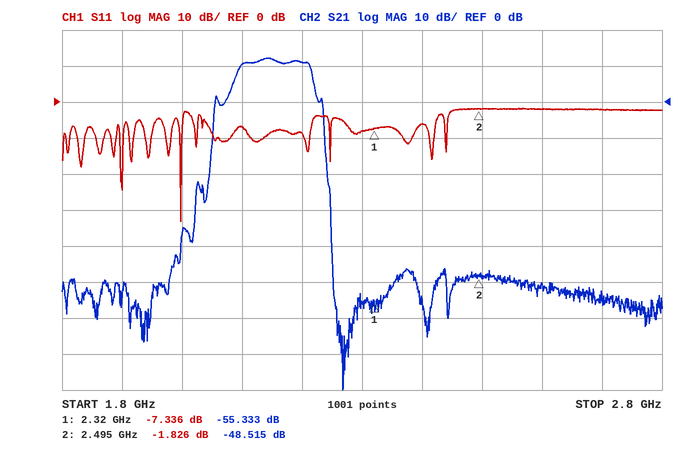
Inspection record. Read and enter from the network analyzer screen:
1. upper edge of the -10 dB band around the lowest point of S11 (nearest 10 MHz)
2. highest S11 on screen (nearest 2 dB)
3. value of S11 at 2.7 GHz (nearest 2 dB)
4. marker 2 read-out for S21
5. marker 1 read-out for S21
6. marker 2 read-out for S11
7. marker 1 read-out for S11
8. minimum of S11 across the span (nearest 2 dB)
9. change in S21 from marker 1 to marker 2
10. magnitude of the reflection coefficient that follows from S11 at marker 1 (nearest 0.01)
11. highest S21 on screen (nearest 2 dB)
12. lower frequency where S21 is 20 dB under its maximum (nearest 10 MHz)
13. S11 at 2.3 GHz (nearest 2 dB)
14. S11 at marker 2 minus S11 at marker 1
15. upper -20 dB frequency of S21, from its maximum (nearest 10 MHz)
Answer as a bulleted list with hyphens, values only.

- 2.00 GHz
- -2 dB
- -2 dB
- -48.515 dB
- -55.333 dB
- -1.826 dB
- -7.336 dB
- -34 dB
- 6.818 dB
- 0.43
- 12 dB
- 2.05 GHz
- -8 dB
- 5.510 dB
- 2.24 GHz
